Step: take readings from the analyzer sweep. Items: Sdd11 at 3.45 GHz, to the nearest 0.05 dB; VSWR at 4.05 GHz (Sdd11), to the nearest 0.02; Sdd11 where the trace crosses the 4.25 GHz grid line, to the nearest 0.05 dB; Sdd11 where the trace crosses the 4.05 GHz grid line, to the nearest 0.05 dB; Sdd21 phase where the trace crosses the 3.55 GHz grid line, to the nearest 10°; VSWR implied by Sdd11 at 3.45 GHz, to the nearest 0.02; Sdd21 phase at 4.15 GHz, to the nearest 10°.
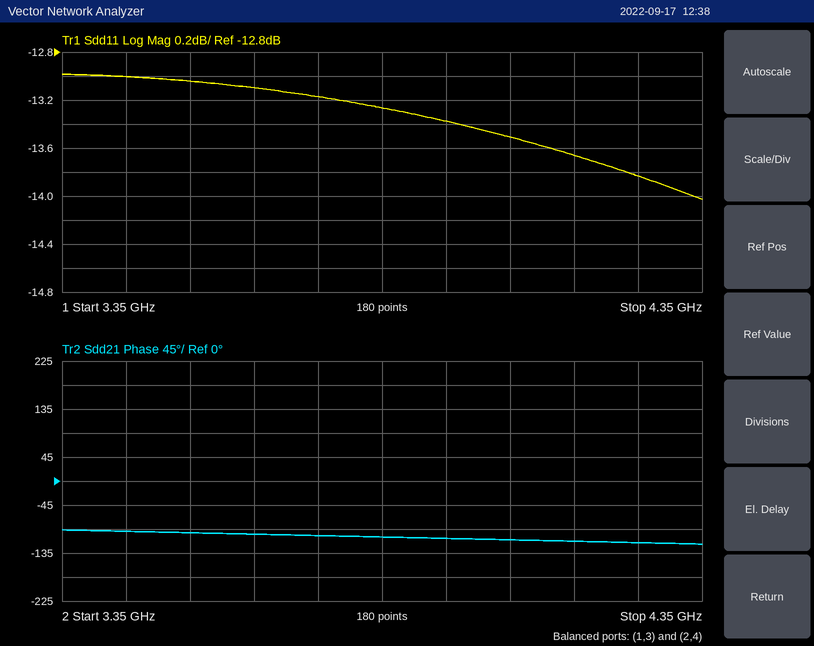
-13.00 dB
1.54
-13.85 dB
-13.50 dB
-100°
1.58
-110°
